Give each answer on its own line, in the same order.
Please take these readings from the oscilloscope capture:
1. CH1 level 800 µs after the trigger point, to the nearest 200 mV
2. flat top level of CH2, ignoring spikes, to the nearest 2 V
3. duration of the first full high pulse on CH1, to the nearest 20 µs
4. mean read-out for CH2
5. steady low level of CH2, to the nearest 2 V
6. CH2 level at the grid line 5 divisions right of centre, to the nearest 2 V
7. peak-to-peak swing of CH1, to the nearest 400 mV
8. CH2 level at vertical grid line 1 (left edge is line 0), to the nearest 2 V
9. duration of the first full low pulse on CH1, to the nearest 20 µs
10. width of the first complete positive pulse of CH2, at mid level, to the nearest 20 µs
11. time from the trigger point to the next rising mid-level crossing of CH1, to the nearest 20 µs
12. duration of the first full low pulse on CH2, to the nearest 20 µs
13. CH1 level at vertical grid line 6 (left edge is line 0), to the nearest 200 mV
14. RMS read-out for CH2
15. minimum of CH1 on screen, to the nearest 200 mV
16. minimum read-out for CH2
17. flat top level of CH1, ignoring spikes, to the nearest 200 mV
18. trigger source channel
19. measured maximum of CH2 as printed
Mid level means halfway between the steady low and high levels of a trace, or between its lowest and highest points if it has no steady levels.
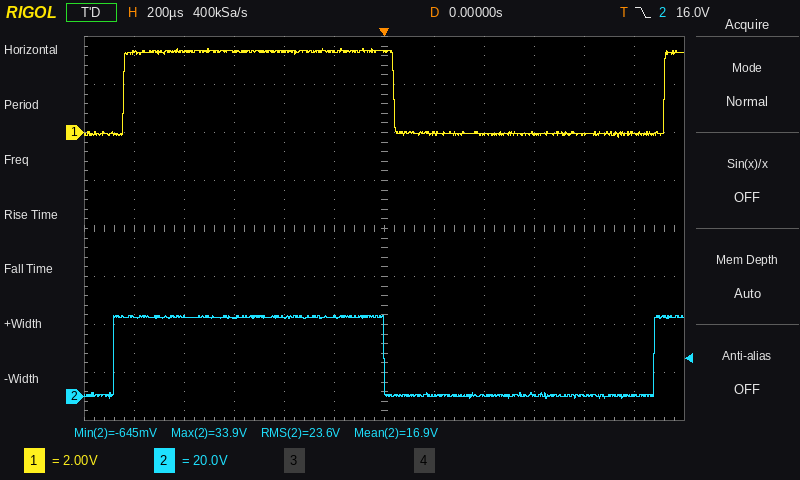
0.0 V
34 V
1.08 ms
16.9 V
0 V
0 V
3.6 V
34 V
1.08 ms
1.08 ms
1.12 ms
1.08 ms
3.4 V
23.6 V
-200 mV
-645 mV
3.4 V
CH2
33.9 V
